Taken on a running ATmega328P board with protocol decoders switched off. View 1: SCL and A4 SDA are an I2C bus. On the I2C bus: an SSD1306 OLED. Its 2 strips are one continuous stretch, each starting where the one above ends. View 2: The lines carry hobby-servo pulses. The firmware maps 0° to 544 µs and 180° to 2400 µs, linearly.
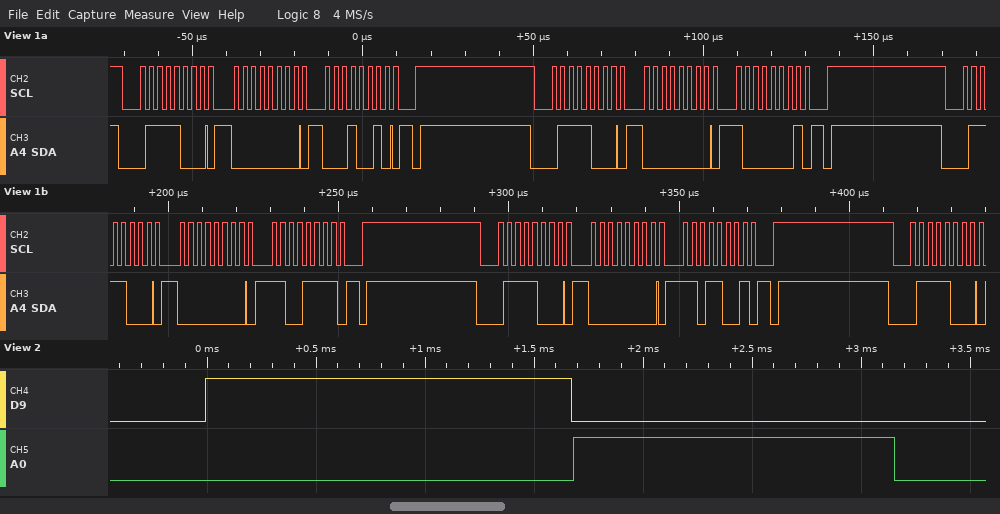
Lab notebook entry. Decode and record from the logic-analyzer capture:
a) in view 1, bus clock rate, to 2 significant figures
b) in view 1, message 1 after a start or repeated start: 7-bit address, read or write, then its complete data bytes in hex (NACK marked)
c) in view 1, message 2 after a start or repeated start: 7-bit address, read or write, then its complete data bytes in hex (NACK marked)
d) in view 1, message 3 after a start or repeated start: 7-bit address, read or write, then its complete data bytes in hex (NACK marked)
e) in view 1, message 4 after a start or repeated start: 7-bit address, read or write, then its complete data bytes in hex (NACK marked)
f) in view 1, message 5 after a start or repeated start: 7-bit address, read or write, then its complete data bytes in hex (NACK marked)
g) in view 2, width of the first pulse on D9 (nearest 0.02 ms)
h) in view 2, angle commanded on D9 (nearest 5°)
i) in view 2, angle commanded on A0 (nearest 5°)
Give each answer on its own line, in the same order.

400 kHz
0x3C write: 00 12
0x3C write: 00 81
0x3C write: 00 CF
0x3C write: 00 D9
0x3C write
1.68 ms
110°
90°
